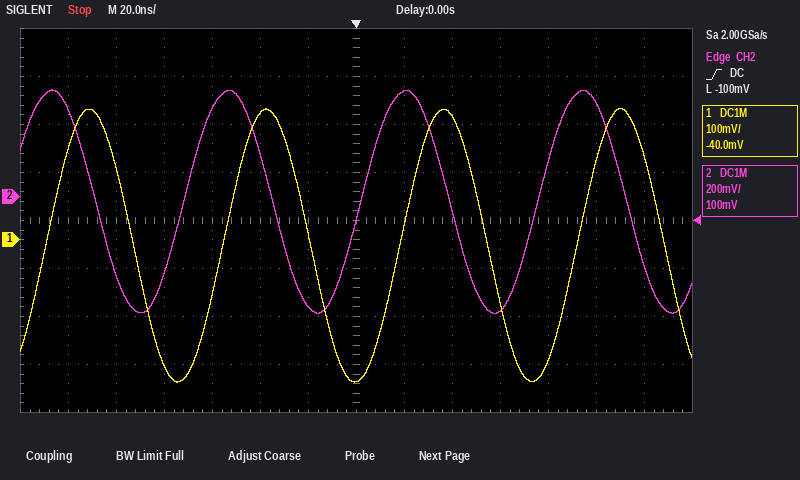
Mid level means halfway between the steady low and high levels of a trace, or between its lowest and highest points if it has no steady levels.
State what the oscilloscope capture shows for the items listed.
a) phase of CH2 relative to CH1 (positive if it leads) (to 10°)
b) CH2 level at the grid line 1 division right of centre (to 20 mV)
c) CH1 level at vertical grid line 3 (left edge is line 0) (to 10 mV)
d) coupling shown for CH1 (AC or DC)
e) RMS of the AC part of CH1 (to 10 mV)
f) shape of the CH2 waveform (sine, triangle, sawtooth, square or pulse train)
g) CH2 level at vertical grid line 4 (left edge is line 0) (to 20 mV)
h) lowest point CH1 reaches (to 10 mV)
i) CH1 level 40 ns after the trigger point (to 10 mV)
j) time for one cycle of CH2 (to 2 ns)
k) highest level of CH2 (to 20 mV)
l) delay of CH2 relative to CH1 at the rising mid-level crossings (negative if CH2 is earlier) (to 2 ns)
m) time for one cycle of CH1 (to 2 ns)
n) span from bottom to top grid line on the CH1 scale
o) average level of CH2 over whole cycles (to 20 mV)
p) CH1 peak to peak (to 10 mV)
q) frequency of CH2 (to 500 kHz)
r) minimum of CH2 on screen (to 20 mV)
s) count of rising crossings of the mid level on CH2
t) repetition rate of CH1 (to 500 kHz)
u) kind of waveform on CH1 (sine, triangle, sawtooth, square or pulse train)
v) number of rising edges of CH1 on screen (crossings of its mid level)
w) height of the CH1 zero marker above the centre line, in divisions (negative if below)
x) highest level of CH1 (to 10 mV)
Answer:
+80°
440 mV
-260 mV
DC
200 mV
sine
360 mV
-300 mV
260 mV
74 ns
440 mV
-16 ns
74 ns
800 mV
-20 mV
570 mV
13.5 MHz
-480 mV
3
13.5 MHz
sine
4
-0.4 div
270 mV
